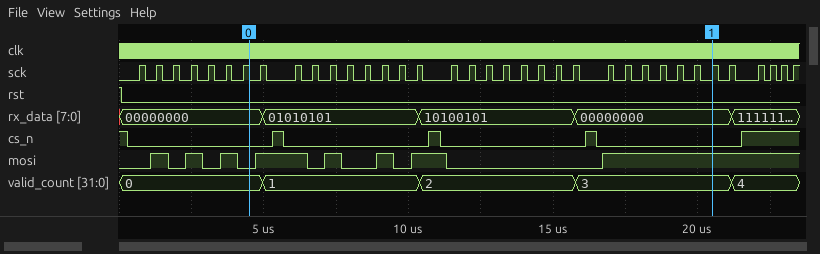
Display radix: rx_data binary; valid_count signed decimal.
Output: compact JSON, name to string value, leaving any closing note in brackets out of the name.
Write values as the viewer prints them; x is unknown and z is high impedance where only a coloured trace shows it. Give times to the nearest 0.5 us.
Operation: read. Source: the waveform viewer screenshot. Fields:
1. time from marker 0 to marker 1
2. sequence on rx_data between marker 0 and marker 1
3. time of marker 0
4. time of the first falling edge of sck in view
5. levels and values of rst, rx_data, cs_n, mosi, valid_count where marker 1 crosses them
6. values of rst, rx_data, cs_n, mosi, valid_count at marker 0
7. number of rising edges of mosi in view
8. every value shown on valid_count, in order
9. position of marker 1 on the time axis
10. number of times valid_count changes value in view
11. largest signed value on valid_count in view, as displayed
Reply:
{"time from marker 0 to marker 1": "16 us", "sequence on rx_data between marker 0 and marker 1": "00000000, 01010101, 10100101, 00000000", "time of marker 0": "4.5 us", "time of the first falling edge of sck in view": "1 us", "levels and values of rst, rx_data, cs_n, mosi, valid_count where marker 1 crosses them": "rst=0, rx_data=00000000, cs_n=0, mosi=1, valid_count=3", "values of rst, rx_data, cs_n, mosi, valid_count at marker 0": "rst=0, rx_data=00000000, cs_n=0, mosi=0, valid_count=0", "number of rising edges of mosi in view": "8", "every value shown on valid_count, in order": "0, 1, 2, 3, 4", "position of marker 1 on the time axis": "20.5 us", "number of times valid_count changes value in view": "4", "largest signed value on valid_count in view, as displayed": "4"}
